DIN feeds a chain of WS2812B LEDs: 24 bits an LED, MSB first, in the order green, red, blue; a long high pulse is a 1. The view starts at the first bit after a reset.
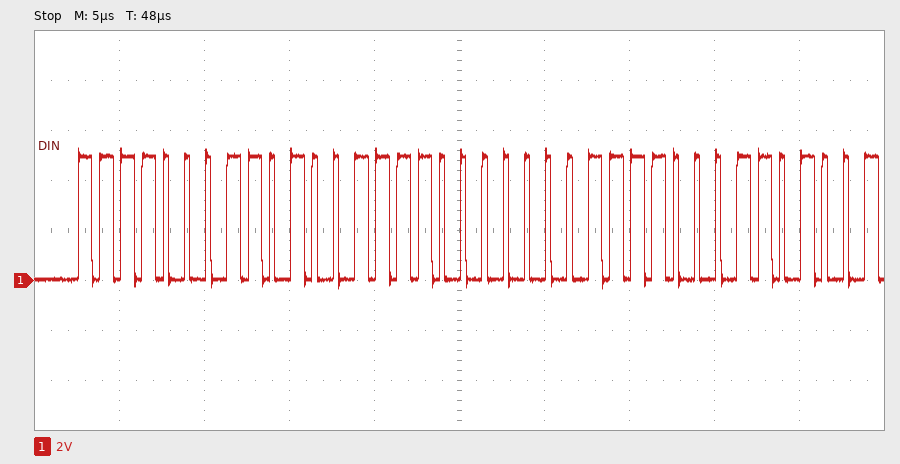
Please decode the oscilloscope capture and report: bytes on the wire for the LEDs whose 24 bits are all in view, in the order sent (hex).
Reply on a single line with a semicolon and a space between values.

F1 A7 80
